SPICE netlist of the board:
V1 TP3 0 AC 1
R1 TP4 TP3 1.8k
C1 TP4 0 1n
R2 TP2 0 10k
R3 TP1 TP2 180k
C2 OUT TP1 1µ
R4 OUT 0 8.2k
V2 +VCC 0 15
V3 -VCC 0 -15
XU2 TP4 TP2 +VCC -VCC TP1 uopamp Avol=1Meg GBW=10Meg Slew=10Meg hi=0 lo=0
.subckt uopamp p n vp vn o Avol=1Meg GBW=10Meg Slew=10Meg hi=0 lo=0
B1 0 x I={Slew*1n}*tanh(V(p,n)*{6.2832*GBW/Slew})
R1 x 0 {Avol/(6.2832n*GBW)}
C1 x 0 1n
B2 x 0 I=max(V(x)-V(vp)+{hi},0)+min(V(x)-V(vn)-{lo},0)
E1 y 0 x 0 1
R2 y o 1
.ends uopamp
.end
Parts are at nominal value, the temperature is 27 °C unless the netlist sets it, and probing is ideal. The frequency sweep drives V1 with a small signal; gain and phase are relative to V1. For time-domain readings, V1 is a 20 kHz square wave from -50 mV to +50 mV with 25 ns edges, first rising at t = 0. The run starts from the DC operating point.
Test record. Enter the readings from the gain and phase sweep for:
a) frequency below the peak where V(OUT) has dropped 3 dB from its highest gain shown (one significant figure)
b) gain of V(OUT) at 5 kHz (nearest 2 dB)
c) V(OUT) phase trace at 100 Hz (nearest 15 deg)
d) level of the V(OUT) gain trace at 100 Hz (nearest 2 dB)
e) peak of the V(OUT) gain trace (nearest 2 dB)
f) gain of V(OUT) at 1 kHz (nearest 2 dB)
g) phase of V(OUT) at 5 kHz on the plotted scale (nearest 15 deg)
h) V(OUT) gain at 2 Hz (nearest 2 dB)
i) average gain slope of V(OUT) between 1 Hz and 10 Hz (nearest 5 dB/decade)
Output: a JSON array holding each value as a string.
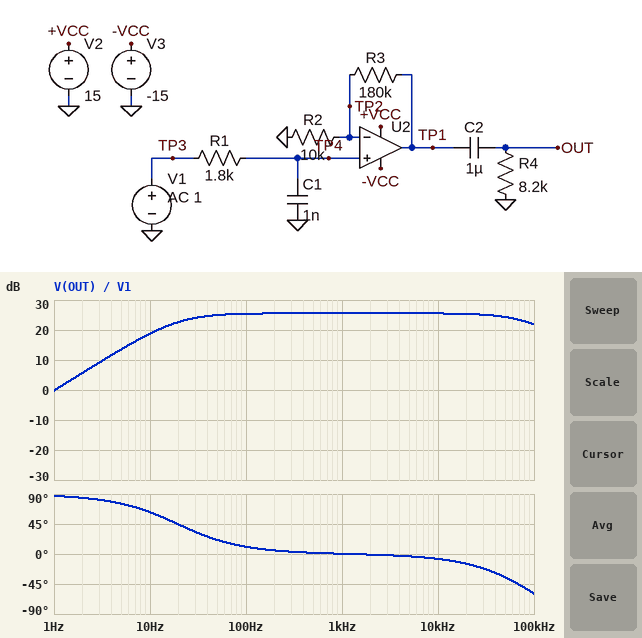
["20 Hz", "26 dB", "15 deg", "26 dB", "26 dB", "26 dB", "0 deg", "6 dB", "20 dB/decade"]
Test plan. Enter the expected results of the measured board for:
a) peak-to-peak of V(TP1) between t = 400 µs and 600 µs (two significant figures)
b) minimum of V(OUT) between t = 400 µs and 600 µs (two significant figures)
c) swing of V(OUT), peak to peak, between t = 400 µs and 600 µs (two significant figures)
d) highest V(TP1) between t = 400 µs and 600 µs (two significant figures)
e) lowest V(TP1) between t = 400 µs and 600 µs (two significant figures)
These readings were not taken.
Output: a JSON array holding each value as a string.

["1.9 V", "-67 mV", "1.9 V", "950 mV", "-950 mV"]
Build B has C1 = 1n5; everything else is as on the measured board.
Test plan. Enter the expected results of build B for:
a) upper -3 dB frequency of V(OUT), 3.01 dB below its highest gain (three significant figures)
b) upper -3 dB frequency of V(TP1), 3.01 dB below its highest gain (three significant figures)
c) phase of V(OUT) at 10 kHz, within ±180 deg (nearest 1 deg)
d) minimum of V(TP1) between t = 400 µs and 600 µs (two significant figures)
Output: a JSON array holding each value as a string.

["58.3 kHz", "58.2 kHz", "-11 deg", "-950 mV"]
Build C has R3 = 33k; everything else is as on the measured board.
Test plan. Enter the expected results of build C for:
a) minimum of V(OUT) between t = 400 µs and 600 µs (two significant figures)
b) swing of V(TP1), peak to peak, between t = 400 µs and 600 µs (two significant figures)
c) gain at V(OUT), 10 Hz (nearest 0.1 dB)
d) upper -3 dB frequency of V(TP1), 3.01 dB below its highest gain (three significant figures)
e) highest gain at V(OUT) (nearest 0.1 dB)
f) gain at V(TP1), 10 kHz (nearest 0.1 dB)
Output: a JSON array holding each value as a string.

["-15 mV", "430 mV", "5.9 dB", "88.3 kHz", "12.7 dB", "12.6 dB"]
